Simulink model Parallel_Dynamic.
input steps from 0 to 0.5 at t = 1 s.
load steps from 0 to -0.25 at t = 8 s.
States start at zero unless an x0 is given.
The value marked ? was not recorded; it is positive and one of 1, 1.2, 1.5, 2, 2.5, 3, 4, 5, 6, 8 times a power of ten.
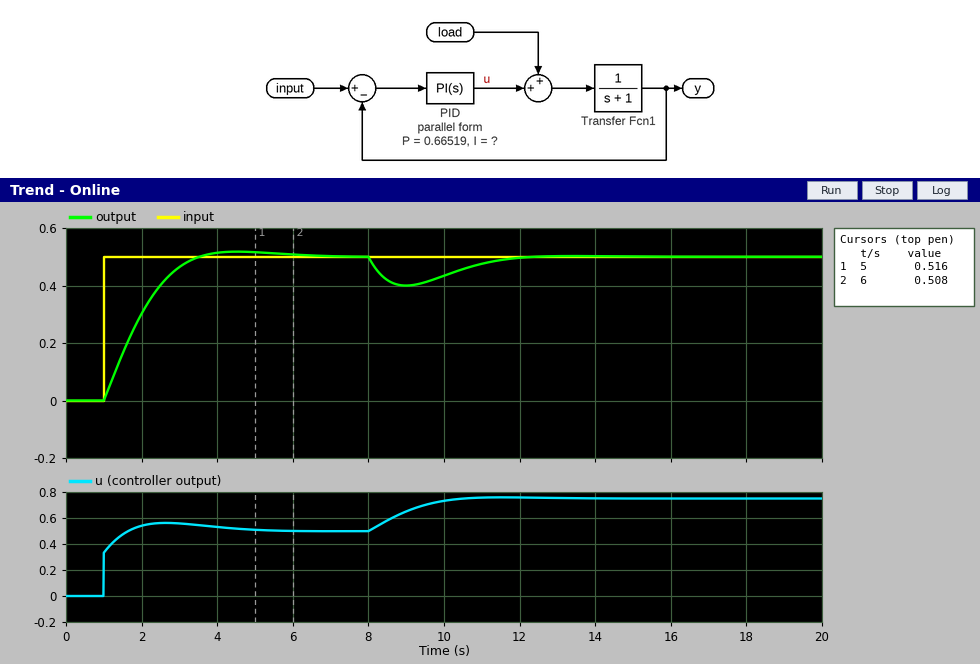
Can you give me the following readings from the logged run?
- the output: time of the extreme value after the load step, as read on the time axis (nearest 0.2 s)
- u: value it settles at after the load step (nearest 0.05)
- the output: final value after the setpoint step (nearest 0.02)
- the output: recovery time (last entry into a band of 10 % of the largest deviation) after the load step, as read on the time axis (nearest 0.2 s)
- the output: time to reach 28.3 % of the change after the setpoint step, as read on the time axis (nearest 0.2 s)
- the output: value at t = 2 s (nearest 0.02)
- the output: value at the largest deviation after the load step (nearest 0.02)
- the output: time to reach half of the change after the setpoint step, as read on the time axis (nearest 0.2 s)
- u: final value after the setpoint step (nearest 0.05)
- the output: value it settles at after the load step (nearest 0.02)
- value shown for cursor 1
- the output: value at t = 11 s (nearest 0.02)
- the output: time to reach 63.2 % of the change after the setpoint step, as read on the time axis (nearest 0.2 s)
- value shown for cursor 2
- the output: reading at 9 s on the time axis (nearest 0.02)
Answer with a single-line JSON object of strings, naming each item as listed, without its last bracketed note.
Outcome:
{"the output: time of the extreme value after the load step, as read on the time axis": "9.0 s", "u: value it settles at after the load step": "0.75", "the output: final value after the setpoint step": "0.50", "the output: recovery time (last entry into a band of 10 % of the largest deviation) after the load step, as read on the time axis": "11.6 s", "the output: time to reach 28.3 % of the change after the setpoint step, as read on the time axis": "1.4 s", "the output: value at t = 2 s": "0.30", "the output: value at the largest deviation after the load step": "0.40", "the output: time to reach half of the change after the setpoint step, as read on the time axis": "1.8 s", "u: final value after the setpoint step": "0.50", "the output: value it settles at after the load step": "0.50", "value shown for cursor 1": "0.516", "the output: value at t = 11 s": "0.48", "the output: time to reach 63.2 % of the change after the setpoint step, as read on the time axis": "2.0 s", "value shown for cursor 2": "0.508", "the output: reading at 9 s on the time axis": "0.40"}
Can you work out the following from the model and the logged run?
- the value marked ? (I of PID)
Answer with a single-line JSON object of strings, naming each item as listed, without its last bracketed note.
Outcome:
{"the value marked ?": "1.2"}
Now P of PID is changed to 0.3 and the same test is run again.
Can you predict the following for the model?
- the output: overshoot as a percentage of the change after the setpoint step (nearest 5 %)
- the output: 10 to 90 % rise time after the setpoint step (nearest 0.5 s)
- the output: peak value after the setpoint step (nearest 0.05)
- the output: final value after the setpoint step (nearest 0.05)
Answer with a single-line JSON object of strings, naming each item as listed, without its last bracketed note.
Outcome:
{"the output: overshoot as a percentage of the change after the setpoint step": "10 %", "the output: 10 to 90 % rise time after the setpoint step": "1.5 s", "the output: peak value after the setpoint step": "0.55", "the output: final value after the setpoint step": "0.50"}
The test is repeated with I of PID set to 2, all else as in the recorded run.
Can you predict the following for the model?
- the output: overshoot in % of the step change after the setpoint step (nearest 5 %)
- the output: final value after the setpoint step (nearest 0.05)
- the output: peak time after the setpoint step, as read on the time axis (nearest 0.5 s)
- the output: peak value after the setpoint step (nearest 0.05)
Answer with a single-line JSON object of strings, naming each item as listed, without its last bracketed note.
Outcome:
{"the output: overshoot in % of the step change after the setpoint step": "10 %", "the output: final value after the setpoint step": "0.50", "the output: peak time after the setpoint step, as read on the time axis": "3.5 s", "the output: peak value after the setpoint step": "0.55"}
